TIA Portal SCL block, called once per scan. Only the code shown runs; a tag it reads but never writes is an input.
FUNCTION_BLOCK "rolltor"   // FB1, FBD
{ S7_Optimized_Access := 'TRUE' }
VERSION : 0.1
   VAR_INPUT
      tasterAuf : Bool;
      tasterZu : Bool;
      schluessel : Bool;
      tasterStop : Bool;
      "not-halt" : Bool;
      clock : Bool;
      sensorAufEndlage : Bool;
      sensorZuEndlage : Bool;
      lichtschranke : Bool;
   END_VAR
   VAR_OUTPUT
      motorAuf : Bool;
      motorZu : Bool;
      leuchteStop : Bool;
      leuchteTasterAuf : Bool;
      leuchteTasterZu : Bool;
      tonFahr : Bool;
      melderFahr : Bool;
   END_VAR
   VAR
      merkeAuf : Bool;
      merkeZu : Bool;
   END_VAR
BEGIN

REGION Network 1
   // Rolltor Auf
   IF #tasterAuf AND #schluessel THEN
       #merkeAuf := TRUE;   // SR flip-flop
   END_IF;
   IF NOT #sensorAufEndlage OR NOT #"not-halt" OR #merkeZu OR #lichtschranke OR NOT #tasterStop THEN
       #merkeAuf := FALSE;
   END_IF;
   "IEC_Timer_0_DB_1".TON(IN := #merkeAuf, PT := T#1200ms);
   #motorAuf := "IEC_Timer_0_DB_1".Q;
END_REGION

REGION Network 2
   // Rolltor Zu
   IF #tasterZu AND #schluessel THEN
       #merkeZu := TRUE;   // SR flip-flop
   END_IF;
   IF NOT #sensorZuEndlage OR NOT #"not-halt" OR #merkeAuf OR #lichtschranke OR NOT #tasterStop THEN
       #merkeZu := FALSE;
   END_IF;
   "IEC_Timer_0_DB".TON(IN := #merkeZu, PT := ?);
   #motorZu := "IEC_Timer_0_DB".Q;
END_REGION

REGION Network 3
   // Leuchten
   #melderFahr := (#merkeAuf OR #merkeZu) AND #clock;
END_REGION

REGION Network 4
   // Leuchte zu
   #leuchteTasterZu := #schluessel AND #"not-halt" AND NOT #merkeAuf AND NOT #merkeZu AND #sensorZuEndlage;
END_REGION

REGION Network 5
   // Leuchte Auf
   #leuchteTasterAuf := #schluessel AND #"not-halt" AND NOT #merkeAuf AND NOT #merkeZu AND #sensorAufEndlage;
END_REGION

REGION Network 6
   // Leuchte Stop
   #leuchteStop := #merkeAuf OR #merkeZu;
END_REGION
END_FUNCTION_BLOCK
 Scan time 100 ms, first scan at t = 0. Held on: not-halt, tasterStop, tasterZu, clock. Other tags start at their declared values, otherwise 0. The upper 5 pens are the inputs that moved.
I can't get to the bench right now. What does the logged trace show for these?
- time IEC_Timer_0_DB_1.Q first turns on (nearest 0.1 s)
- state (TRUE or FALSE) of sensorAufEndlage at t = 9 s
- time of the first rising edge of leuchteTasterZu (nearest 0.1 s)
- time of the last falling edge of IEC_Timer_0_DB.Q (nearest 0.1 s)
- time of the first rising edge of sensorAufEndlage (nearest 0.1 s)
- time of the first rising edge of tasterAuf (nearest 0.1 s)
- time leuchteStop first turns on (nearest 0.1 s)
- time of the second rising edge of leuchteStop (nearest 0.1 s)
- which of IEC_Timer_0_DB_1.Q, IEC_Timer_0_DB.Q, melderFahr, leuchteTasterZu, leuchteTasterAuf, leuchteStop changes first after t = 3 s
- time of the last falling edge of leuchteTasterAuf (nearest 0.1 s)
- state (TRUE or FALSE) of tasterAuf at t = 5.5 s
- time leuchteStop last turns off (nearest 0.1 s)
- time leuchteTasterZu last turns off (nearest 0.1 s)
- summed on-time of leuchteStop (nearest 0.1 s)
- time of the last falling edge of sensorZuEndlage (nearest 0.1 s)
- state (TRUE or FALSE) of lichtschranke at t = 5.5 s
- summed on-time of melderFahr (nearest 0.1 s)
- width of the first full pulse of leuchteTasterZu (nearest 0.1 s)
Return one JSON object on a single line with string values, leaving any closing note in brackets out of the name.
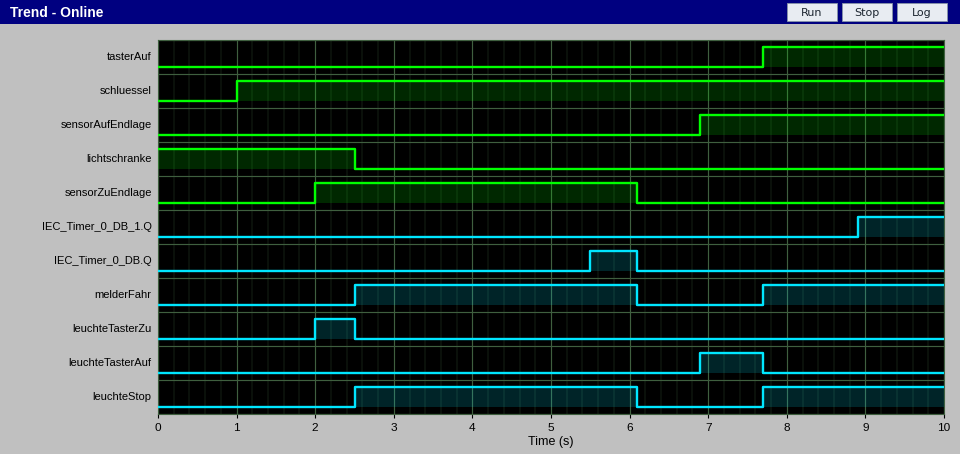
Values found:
{"time IEC_Timer_0_DB_1.Q first turns on": "8.9 s", "state (TRUE or FALSE) of sensorAufEndlage at t = 9 s": "TRUE", "time of the first rising edge of leuchteTasterZu": "2.0 s", "time of the last falling edge of IEC_Timer_0_DB.Q": "6.1 s", "time of the first rising edge of sensorAufEndlage": "6.9 s", "time of the first rising edge of tasterAuf": "7.7 s", "time leuchteStop first turns on": "2.5 s", "time of the second rising edge of leuchteStop": "7.7 s", "which of IEC_Timer_0_DB_1.Q, IEC_Timer_0_DB.Q, melderFahr, leuchteTasterZu, leuchteTasterAuf, leuchteStop changes first after t = 3 s": "IEC_Timer_0_DB.Q", "time of the last falling edge of leuchteTasterAuf": "7.7 s", "state (TRUE or FALSE) of tasterAuf at t = 5.5 s": "FALSE", "time leuchteStop last turns off": "6.1 s", "time leuchteTasterZu last turns off": "2.5 s", "summed on-time of leuchteStop": "5.9 s", "time of the last falling edge of sensorZuEndlage": "6.1 s", "state (TRUE or FALSE) of lichtschranke at t = 5.5 s": "FALSE", "summed on-time of melderFahr": "5.9 s", "width of the first full pulse of leuchteTasterZu": "0.5 s"}
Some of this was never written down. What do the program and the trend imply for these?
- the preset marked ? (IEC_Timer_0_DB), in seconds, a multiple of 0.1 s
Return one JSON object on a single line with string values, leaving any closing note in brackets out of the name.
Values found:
{"the preset marked ? (IEC_Timer_0_DB), in seconds, a multiple of 0.1 s": "3.0 s"}
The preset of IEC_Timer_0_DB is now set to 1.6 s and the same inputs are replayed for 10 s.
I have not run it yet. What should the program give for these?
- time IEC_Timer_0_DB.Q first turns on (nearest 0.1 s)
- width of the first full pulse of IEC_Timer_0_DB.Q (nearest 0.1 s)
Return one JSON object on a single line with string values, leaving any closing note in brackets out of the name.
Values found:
{"time IEC_Timer_0_DB.Q first turns on": "4.1 s", "width of the first full pulse of IEC_Timer_0_DB.Q": "2.0 s"}
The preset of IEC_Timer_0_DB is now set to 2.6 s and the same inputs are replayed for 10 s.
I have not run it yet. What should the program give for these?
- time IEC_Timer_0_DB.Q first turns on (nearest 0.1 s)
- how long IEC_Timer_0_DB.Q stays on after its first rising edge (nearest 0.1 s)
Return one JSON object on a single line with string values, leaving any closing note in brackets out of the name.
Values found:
{"time IEC_Timer_0_DB.Q first turns on": "5.1 s", "how long IEC_Timer_0_DB.Q stays on after its first rising edge": "1.0 s"}
